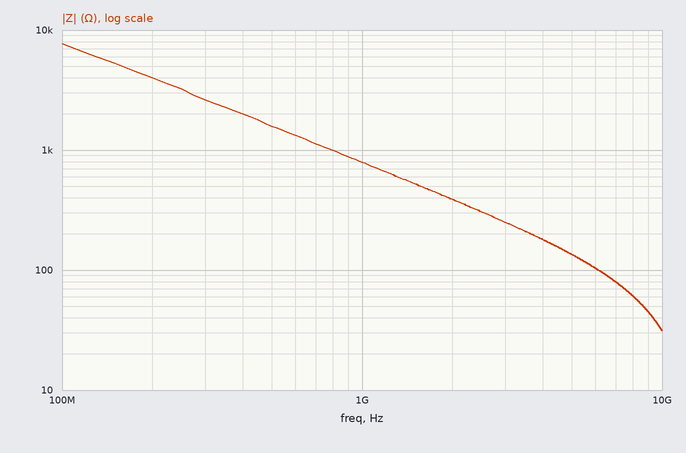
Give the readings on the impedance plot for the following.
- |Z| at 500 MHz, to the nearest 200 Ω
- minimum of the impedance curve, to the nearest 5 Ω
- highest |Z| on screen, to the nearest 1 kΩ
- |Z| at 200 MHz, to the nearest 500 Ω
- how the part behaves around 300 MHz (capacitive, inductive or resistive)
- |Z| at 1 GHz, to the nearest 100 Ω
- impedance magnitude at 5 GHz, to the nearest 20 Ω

1.6 kΩ
30 Ω
8 kΩ
4.0 kΩ
capacitive
800 Ω
140 Ω
